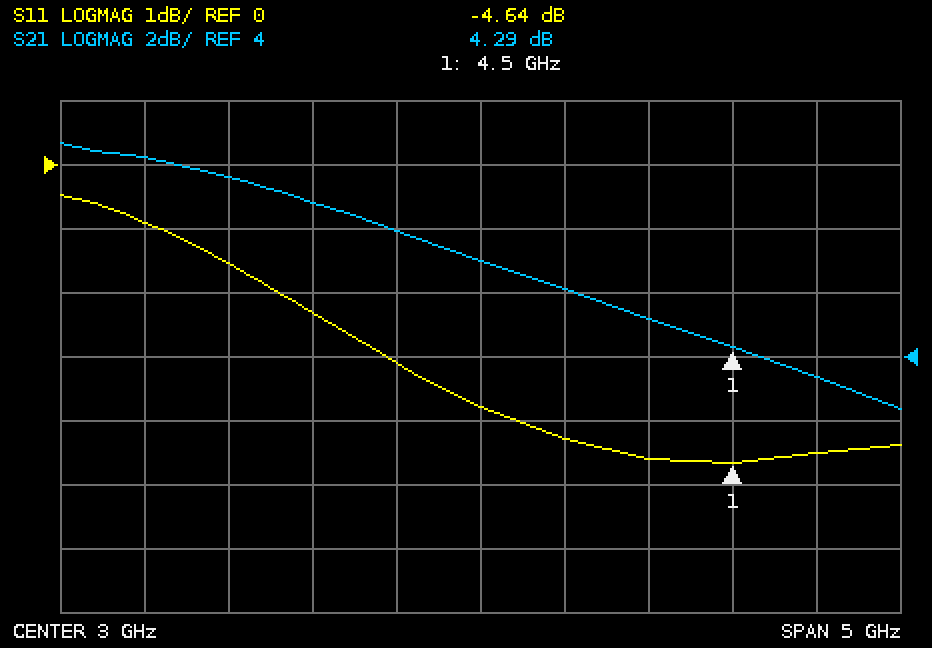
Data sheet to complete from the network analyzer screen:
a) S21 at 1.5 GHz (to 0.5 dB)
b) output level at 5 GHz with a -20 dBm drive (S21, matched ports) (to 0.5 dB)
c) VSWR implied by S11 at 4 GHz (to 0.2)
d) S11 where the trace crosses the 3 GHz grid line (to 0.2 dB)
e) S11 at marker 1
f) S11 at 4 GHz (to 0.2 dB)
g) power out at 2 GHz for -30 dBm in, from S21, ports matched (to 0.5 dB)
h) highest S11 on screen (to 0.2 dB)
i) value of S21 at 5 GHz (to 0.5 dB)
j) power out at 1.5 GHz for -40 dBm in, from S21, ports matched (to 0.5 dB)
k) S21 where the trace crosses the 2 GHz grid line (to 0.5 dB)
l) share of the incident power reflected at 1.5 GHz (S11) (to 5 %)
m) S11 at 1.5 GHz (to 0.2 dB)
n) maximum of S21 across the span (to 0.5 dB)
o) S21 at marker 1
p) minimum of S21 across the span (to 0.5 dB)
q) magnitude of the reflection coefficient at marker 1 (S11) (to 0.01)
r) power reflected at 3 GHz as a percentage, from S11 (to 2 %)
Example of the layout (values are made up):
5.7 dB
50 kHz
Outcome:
9.5 dB
-16.5 dBm
3.8
-3.8 dB
-4.64 dB
-4.6 dB
-21.0 dBm
-0.4 dB
3.5 dB
-30.5 dBm
9.0 dB
70 %
-1.6 dB
10.5 dB
4.29 dB
2.5 dB
0.59
42 %
